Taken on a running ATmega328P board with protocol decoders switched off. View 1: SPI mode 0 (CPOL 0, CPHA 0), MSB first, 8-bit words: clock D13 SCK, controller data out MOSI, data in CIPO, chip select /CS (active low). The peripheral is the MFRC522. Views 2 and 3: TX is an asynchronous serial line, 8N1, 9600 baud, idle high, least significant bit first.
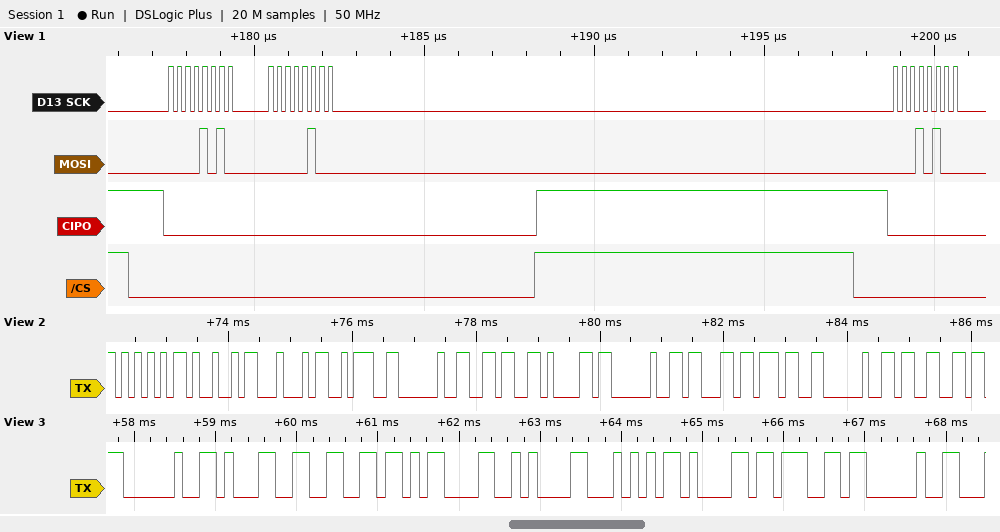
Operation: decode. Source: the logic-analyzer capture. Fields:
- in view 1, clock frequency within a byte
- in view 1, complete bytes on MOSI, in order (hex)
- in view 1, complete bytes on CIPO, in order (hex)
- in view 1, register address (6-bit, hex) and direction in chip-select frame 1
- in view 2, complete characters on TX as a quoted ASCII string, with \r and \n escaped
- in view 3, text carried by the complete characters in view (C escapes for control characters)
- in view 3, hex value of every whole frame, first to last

4 MHz
0x0A 0x04 0x14
0x00 0x00 0x00
0x05 write
"UID: 6a c7 3"
" 1f\r\nTag "
20 31 66 0D 0A 54 61 67 20
